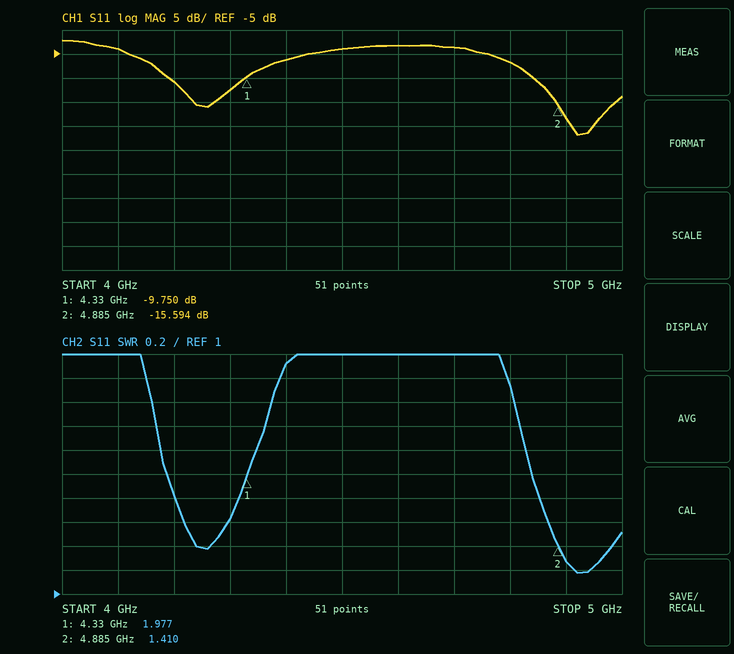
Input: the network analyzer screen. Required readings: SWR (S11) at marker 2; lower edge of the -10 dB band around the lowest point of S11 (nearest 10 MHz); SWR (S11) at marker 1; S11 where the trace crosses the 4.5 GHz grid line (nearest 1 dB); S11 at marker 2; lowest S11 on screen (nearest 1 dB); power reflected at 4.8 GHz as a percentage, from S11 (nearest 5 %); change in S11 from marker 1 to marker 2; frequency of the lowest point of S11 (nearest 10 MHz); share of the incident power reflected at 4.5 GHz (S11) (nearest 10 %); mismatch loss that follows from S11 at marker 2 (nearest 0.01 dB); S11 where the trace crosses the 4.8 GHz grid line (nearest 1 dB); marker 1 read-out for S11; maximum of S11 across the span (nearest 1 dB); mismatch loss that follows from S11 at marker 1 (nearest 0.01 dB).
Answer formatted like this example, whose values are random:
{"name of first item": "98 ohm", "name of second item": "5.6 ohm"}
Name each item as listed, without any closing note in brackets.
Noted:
{"SWR (S11) at marker 2": "1.410", "lower edge of the -10 dB band around the lowest point of S11": "4.84 GHz", "SWR (S11) at marker 1": "1.977", "S11 where the trace crosses the 4.5 GHz grid line": "-4 dB", "S11 at marker 2": "-15.594 dB", "lowest S11 on screen": "-22 dB", "power reflected at 4.8 GHz as a percentage, from S11": "20 %", "change in S11 from marker 1 to marker 2": "-5.844 dB", "frequency of the lowest point of S11": "4.92 GHz", "share of the incident power reflected at 4.5 GHz (S11)": "40 %", "mismatch loss that follows from S11 at marker 2": "0.12 dB", "S11 where the trace crosses the 4.8 GHz grid line": "-7 dB", "marker 1 read-out for S11": "-9.750 dB", "maximum of S11 across the span": "-2 dB", "mismatch loss that follows from S11 at marker 1": "0.49 dB"}
